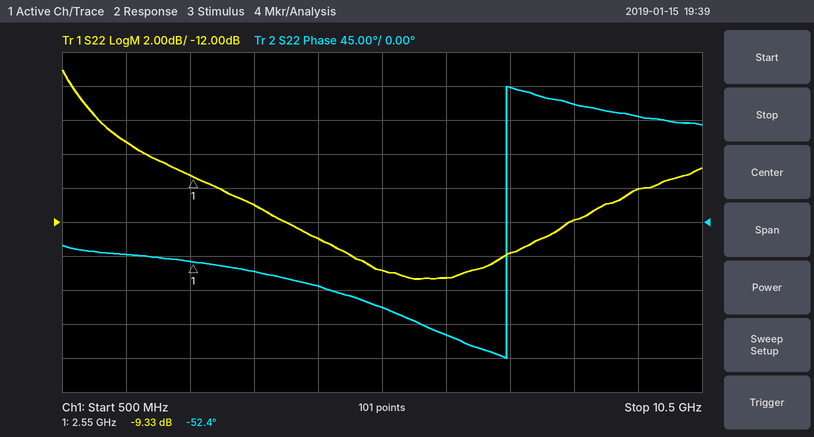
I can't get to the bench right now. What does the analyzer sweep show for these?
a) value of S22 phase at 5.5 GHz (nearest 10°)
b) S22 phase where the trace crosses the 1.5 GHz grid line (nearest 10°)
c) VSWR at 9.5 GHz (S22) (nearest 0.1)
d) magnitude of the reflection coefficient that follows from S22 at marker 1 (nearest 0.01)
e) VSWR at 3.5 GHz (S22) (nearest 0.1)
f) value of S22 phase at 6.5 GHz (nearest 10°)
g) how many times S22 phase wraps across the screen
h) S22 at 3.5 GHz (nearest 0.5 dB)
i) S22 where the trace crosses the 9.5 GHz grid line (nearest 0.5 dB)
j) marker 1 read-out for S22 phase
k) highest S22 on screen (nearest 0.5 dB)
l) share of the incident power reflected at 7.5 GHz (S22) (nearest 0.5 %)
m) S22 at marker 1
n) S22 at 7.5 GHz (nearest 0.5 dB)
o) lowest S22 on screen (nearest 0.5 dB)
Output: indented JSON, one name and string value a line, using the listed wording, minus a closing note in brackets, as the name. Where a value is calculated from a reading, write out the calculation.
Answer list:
{
  "value of S22 phase at 5.5 GHz": "-110°",
  "S22 phase where the trace crosses the 1.5 GHz grid line": "-40°",
  "VSWR at 9.5 GHz (S22)": "|Γ| = 10^(-10/20) = 0.3162; VSWR = (1 + 0.3162)/(1 − 0.3162) ≈ 1.9",
  "magnitude of the reflection coefficient that follows from S22 at marker 1": "10^(-9.33/20) ≈ 0.34",
  "VSWR at 3.5 GHz (S22)": "|Γ| = 10^(-11/20) = 0.2818; VSWR = (1 + 0.2818)/(1 − 0.2818) ≈ 1.8",
  "value of S22 phase at 6.5 GHz": "-150°",
  "how many times S22 phase wraps across the screen": "1",
  "S22 at 3.5 GHz": "-11.0 dB",
  "S22 where the trace crosses the 9.5 GHz grid line": "-10.0 dB",
  "marker 1 read-out for S22 phase": "-52.4°",
  "highest S22 on screen": "-3.0 dB",
  "share of the incident power reflected at 7.5 GHz (S22)": "10^(-14/10) ≈ 4.0 %",
  "S22 at marker 1": "-9.33 dB",
  "S22 at 7.5 GHz": "-14.0 dB",
  "lowest S22 on screen": "-15.5 dB"
}
